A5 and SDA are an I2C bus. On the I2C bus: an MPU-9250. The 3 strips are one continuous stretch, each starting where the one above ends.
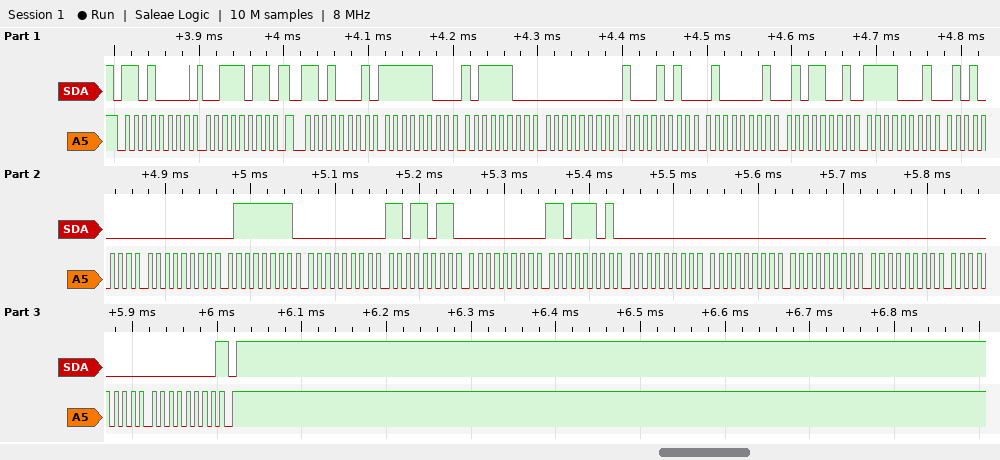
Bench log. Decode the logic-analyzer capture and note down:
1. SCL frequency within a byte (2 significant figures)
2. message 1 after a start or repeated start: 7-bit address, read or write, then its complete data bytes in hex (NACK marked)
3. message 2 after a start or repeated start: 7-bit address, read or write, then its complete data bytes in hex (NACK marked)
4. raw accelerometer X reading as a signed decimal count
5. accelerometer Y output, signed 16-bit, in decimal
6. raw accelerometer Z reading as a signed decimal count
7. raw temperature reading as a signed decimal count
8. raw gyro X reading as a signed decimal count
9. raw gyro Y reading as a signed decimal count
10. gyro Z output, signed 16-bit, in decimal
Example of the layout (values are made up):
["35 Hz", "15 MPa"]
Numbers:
["100 kHz", "0x68 write: 3B", "0x68 read: FC BC 00 8A 41 59 F1 50 00 7F 00 DB 00 DD 00 00 00 00 00 00 NACK", "-836", "138", "16729", "-3760", "127", "219", "221"]
